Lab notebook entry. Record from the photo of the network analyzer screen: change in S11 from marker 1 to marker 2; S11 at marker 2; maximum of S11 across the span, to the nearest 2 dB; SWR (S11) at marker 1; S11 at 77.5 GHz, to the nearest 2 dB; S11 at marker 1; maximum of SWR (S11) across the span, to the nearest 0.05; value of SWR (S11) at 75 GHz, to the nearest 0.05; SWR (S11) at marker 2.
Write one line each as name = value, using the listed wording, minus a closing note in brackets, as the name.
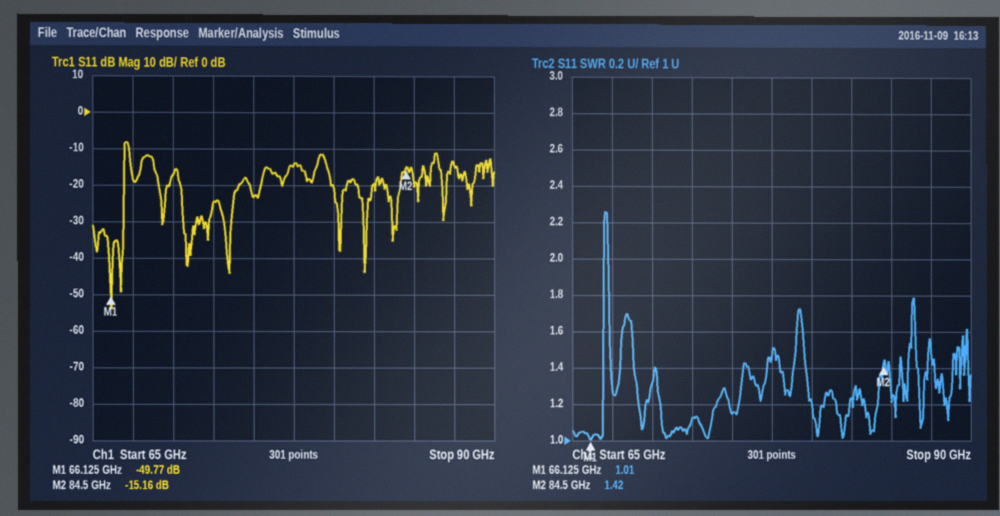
change in S11 from marker 1 to marker 2 = 34.61 dB
S11 at marker 2 = -15.16 dB
maximum of S11 across the span, to the nearest 2 dB = -8 dB
SWR (S11) at marker 1 = 1.01
S11 at 77.5 GHz, to the nearest 2 dB = -14 dB
S11 at marker 1 = -49.77 dB
maximum of SWR (S11) across the span, to the nearest 0.05 = 2.25
value of SWR (S11) at 75 GHz, to the nearest 0.05 = 1.15
SWR (S11) at marker 2 = 1.42
